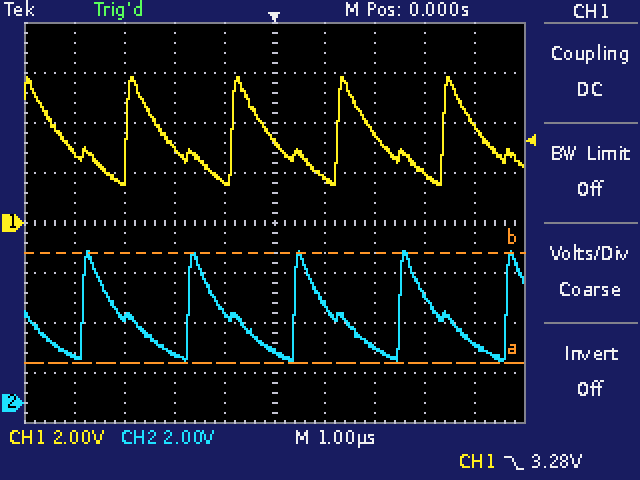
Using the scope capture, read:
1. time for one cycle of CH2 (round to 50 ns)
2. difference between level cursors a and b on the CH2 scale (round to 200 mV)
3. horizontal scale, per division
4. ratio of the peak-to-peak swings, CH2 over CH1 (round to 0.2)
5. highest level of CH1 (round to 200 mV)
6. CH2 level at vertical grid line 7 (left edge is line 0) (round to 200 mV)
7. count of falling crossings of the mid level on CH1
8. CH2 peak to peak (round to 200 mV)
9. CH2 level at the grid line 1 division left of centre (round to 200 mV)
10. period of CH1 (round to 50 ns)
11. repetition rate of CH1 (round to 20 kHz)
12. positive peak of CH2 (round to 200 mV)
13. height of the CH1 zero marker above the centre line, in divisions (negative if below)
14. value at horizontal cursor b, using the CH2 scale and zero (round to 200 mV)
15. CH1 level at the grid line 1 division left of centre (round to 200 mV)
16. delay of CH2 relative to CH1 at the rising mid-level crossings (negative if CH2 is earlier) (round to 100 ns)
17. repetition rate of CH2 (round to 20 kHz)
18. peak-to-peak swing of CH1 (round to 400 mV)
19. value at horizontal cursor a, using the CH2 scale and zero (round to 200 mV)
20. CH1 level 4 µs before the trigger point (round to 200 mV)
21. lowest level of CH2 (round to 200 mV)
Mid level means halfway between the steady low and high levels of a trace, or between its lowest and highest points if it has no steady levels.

2.10 µs
4.4 V
1 µs
1.0
5.8 V
2.2 V
5
4.4 V
3.6 V
2.10 µs
480 kHz
6.0 V
0.0 div
6.0 V
1.6 V
-900 ns
480 kHz
4.4 V
1.6 V
2.8 V
1.6 V
